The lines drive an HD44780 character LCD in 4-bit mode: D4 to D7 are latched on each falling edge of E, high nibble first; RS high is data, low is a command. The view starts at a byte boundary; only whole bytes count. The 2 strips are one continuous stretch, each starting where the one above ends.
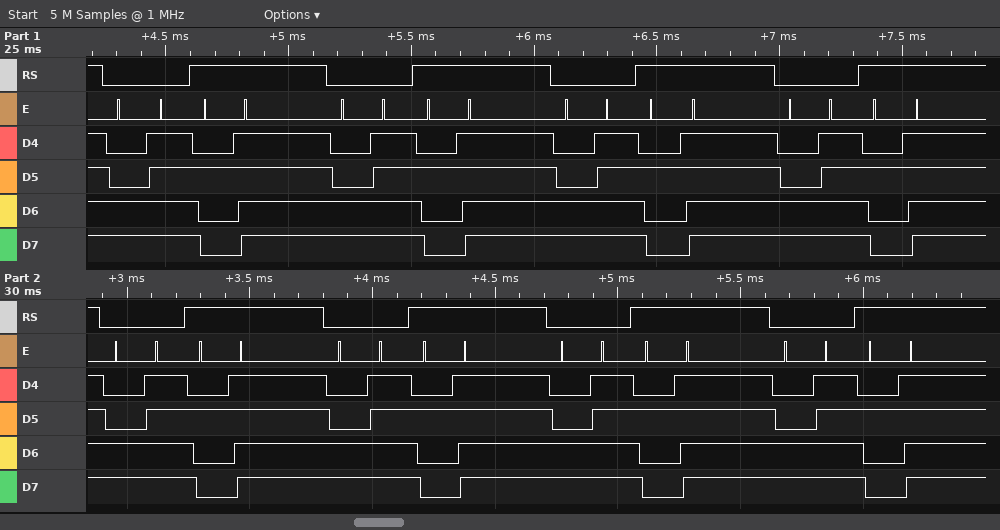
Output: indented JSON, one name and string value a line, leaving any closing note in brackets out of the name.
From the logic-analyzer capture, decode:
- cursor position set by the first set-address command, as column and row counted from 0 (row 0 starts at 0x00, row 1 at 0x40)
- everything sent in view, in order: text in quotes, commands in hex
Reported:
{
  "cursor position set by the first set-address command, as column and row counted from 0": "column 15, row 1",
  "everything sent in view, in order: text in quotes, commands in hex": "0xCF \"/\" 0xCF \"/\" 0xCF \"/\" 0xCF \"/\" 0xCF \"/\" 0xCF \"/\" 0xCF \"/\" 0xCF \"/\""
}
